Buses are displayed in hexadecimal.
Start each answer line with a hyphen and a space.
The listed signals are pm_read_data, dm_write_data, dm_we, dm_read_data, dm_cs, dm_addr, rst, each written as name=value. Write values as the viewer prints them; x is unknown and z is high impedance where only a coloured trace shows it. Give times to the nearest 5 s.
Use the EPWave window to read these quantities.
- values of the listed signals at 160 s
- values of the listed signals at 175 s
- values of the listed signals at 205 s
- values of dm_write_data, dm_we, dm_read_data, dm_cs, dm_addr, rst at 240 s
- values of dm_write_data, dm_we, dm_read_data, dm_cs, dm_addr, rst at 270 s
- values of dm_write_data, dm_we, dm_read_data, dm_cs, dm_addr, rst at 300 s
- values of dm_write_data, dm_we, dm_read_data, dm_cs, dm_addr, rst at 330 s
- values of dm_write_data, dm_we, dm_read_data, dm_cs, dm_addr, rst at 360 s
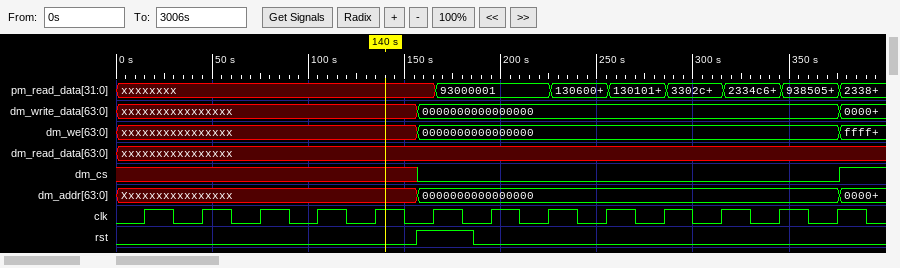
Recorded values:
- pm_read_data=xxxxxxxx, dm_write_data=0000000000000000, dm_we=0000000000000000, dm_read_data=xxxxxxxxxxxxxxxx, dm_cs=0, dm_addr=0000000000000000, rst=1
- pm_read_data=93000001, dm_write_data=0000000000000000, dm_we=0000000000000000, dm_read_data=xxxxxxxxxxxxxxxx, dm_cs=0, dm_addr=0000000000000000, rst=1
- pm_read_data=93000001, dm_write_data=0000000000000000, dm_we=0000000000000000, dm_read_data=xxxxxxxxxxxxxxxx, dm_cs=0, dm_addr=0000000000000000, rst=0
- dm_write_data=0000000000000000, dm_we=0000000000000000, dm_read_data=xxxxxxxxxxxxxxxx, dm_cs=0, dm_addr=0000000000000000, rst=0
- dm_write_data=0000000000000000, dm_we=0000000000000000, dm_read_data=xxxxxxxxxxxxxxxx, dm_cs=0, dm_addr=0000000000000000, rst=0
- dm_write_data=0000000000000000, dm_we=0000000000000000, dm_read_data=xxxxxxxxxxxxxxxx, dm_cs=0, dm_addr=0000000000000000, rst=0
- dm_write_data=0000000000000000, dm_we=0000000000000000, dm_read_data=xxxxxxxxxxxxxxxx, dm_cs=0, dm_addr=0000000000000000, rst=0
- dm_write_data=0000000000000000, dm_we=0000000000000000, dm_read_data=xxxxxxxxxxxxxxxx, dm_cs=0, dm_addr=0000000000000000, rst=0
